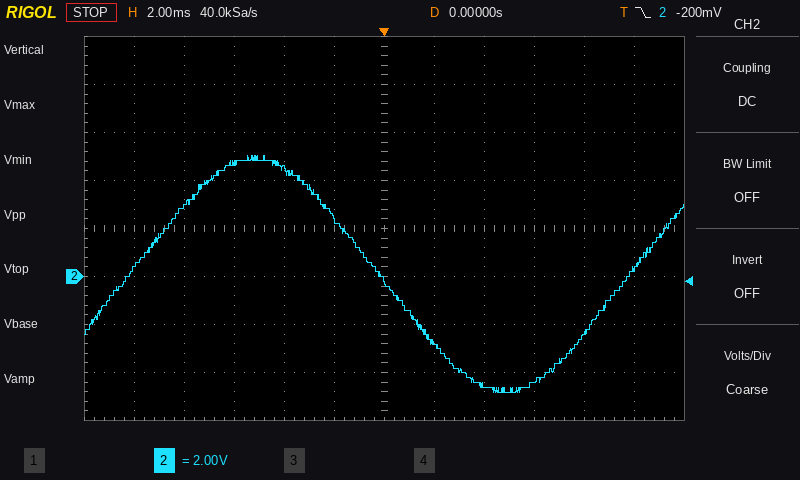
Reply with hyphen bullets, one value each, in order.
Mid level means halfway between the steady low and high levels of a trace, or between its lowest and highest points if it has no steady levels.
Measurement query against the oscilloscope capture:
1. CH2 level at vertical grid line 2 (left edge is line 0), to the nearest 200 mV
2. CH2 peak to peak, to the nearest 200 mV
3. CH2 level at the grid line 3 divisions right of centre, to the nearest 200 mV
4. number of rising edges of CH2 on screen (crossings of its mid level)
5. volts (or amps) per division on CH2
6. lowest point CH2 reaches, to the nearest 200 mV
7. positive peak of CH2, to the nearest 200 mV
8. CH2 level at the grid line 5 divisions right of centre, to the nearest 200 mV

- 3.0 V
- 9.8 V
- -4.4 V
- 2
- 2 V
- -4.8 V
- 5.0 V
- 400 mV
